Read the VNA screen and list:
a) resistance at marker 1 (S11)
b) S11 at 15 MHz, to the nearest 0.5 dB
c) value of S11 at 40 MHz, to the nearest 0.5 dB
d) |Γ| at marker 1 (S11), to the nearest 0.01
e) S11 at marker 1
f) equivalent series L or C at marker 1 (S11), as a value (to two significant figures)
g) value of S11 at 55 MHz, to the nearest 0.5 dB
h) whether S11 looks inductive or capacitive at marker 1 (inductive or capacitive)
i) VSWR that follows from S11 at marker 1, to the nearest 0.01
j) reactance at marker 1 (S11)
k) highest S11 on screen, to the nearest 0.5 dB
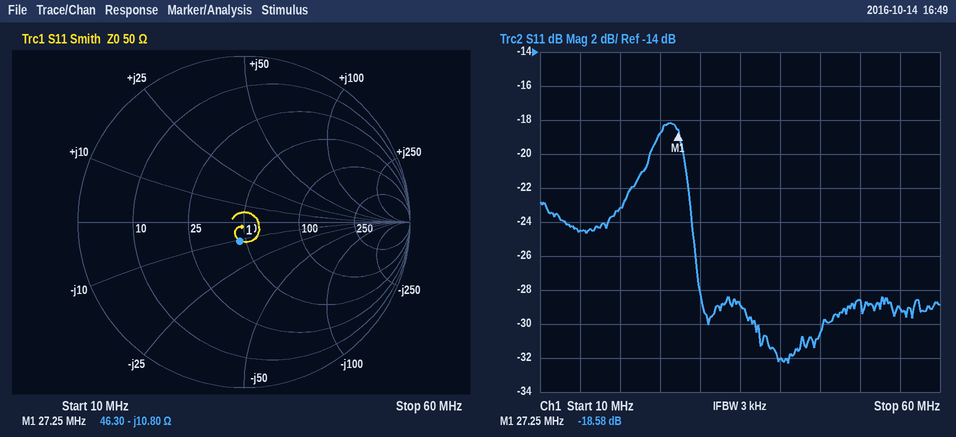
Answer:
46.30 Ω
-24.5 dB
-32.0 dB
0.12
-18.58 dB
540 pF
-29.0 dB
capacitive
1.27
-10.80 Ω
-18.0 dB
